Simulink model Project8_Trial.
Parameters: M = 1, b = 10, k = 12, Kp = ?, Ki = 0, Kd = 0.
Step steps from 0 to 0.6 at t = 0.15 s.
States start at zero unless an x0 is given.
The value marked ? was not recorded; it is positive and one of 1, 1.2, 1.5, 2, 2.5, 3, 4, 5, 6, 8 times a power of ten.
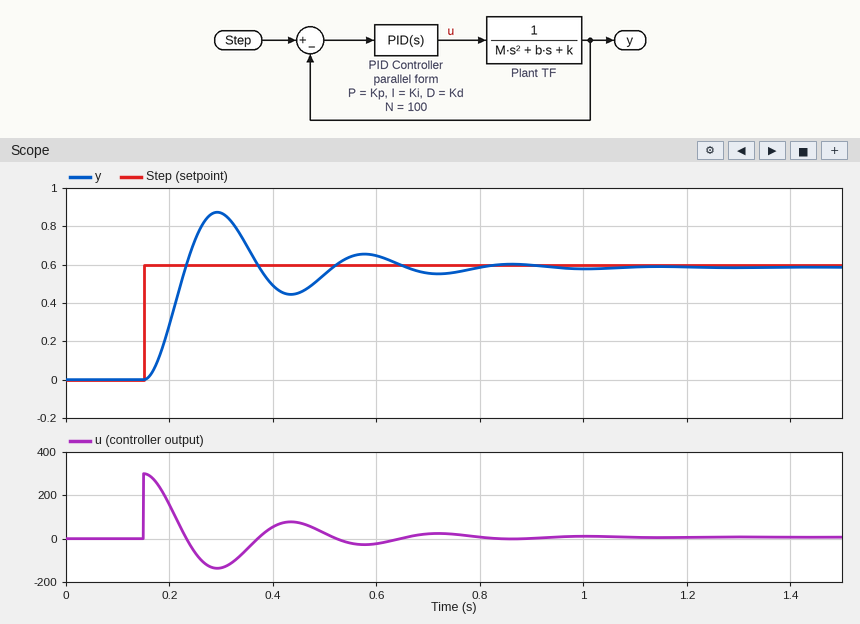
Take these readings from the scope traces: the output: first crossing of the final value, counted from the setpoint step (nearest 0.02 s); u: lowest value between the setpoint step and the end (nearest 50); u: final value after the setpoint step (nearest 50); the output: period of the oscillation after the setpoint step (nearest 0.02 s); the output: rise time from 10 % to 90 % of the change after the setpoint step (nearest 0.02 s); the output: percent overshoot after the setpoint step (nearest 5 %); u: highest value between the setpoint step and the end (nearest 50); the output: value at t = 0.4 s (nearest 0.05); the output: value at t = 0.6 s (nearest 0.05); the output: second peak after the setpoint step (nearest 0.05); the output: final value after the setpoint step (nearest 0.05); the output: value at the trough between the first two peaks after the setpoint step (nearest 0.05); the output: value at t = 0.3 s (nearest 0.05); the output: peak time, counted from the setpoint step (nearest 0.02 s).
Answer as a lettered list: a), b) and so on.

a) 0.08 s
b) -150
c) 0
d) 0.28 s
e) 0.06 s
f) 50 %
g) 300
h) 0.50
i) 0.65
j) 0.65
k) 0.60
l) 0.45
m) 0.85
n) 0.14 s
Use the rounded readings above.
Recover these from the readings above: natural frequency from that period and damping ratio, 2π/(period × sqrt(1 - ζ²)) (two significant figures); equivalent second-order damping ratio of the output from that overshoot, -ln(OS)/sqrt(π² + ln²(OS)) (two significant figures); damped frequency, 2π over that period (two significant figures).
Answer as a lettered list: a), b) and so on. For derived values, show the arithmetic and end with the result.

a) 2π / (0.28 × sqrt(1 - 0.22²)) = 23 rad/s
b) ln(0.5) = -0.693; 0.693 / sqrt(9.870 + 0.480) = 0.22
c) 2π / 0.28 = 22 rad/s
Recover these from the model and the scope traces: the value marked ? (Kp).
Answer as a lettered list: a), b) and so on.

a) 500
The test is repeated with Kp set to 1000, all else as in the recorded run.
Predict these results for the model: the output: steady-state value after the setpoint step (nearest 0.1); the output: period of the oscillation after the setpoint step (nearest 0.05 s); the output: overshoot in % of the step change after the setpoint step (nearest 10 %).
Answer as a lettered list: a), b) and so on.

a) 0.6
b) 0.20 s
c) 60 %
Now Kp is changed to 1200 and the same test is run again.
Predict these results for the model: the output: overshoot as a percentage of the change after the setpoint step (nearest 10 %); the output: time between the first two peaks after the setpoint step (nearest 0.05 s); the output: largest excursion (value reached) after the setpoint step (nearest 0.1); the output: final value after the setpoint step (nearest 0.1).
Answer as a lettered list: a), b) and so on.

a) 60 %
b) 0.20 s
c) 1.0
d) 0.6
